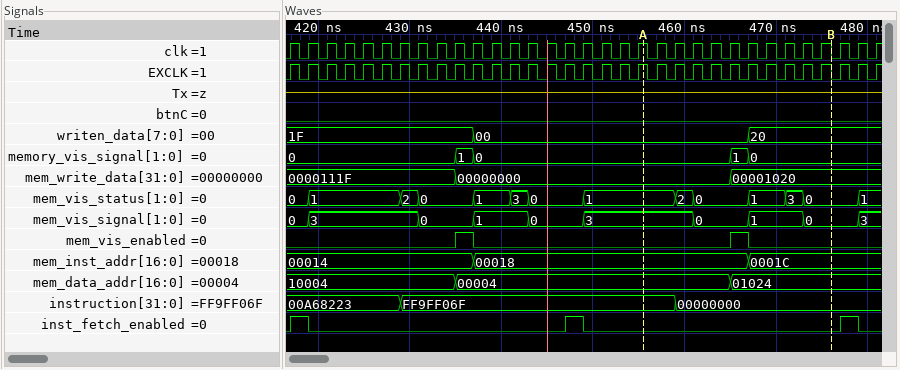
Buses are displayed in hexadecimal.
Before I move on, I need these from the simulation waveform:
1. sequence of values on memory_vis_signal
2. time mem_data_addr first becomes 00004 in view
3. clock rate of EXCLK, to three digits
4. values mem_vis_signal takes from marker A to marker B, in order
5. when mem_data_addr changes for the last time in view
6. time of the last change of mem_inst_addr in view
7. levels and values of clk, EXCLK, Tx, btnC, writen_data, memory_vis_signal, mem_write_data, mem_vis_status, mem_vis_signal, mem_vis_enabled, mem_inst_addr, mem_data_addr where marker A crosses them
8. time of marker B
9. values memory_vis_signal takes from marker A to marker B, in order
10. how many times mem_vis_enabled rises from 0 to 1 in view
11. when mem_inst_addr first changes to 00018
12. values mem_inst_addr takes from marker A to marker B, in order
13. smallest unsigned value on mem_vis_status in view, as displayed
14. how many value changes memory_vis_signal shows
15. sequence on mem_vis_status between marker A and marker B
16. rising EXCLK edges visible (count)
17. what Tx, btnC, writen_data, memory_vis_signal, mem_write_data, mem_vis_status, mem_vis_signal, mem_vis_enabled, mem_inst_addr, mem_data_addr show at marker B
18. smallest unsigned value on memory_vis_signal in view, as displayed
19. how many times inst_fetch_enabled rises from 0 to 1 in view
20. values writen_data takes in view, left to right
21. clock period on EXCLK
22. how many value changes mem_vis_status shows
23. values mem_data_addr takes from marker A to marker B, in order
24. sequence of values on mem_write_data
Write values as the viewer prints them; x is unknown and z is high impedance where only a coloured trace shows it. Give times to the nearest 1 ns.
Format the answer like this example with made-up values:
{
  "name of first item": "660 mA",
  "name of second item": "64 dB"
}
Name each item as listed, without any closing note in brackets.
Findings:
{
  "sequence of values on memory_vis_signal": "0, 1, 0, 1, 0",
  "time mem_data_addr first becomes 00004 in view": "435 ns",
  "clock rate of EXCLK, to three digits": "500 MHz",
  "values mem_vis_signal takes from marker A to marker B, in order": "3, 0, 1, 0",
  "when mem_data_addr changes for the last time in view": "465 ns",
  "time of the last change of mem_inst_addr in view": "467 ns",
  "levels and values of clk, EXCLK, Tx, btnC, writen_data, memory_vis_signal, mem_write_data, mem_vis_status, mem_vis_signal, mem_vis_enabled, mem_inst_addr, mem_data_addr where marker A crosses them": "clk=1, EXCLK=1, Tx=z, btnC=0, writen_data=00, memory_vis_signal=0, mem_write_data=00000000, mem_vis_status=1, mem_vis_signal=3, mem_vis_enabled=0, mem_inst_addr=00018, mem_data_addr=00004",
  "time of marker B": "476 ns",
  "values memory_vis_signal takes from marker A to marker B, in order": "0, 1, 0",
  "how many times mem_vis_enabled rises from 0 to 1 in view": "2",
  "when mem_inst_addr first changes to 00018": "437 ns",
  "values mem_inst_addr takes from marker A to marker B, in order": "00018, 0001C",
  "smallest unsigned value on mem_vis_status in view, as displayed": "0",
  "how many value changes memory_vis_signal shows": "4",
  "sequence on mem_vis_status between marker A and marker B": "1, 2, 0, 1, 3, 0",
  "rising EXCLK edges visible": "33",
  "what Tx, btnC, writen_data, memory_vis_signal, mem_write_data, mem_vis_status, mem_vis_signal, mem_vis_enabled, mem_inst_addr, mem_data_addr show at marker B": "Tx=z, btnC=0, writen_data=20, memory_vis_signal=0, mem_write_data=00001020, mem_vis_status=0, mem_vis_signal=0, mem_vis_enabled=0, mem_inst_addr=0001C, mem_data_addr=01024",
  "smallest unsigned value on memory_vis_signal in view, as displayed": "0",
  "how many times inst_fetch_enabled rises from 0 to 1 in view": "3",
  "values writen_data takes in view, left to right": "1F, 00, 20",
  "clock period on EXCLK": "2 ns",
  "how many value changes mem_vis_status shows": "13",
  "values mem_data_addr takes from marker A to marker B, in order": "00004, 01024",
  "sequence of values on mem_write_data": "0000111F, 00000000, 00001020"
}
